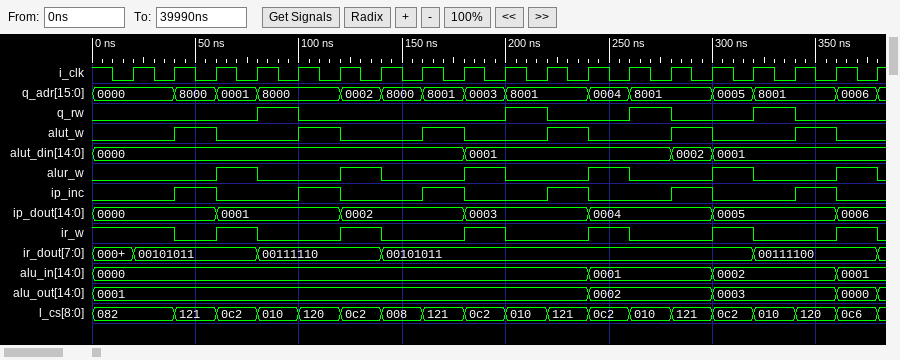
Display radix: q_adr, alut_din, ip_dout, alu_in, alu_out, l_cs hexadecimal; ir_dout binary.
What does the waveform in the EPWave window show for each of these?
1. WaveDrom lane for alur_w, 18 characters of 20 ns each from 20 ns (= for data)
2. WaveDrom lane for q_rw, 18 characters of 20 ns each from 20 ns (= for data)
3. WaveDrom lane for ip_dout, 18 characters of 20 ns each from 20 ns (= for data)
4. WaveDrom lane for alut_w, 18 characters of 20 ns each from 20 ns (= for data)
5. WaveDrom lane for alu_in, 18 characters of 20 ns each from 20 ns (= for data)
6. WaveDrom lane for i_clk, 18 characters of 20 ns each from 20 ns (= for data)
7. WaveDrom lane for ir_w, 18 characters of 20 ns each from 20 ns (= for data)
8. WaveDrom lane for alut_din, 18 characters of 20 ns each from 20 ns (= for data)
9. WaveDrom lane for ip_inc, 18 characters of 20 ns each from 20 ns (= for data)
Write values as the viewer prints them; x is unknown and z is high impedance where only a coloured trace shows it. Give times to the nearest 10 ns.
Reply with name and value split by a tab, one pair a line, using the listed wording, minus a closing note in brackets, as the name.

WaveDrom lane for alur_w, 18 characters of 20 ns each from 20 ns	{name: 'alur_w', wave: '0.10.10.10.10.10.1'}
WaveDrom lane for q_rw, 18 characters of 20 ns each from 20 ns	{name: 'q_rw', wave: '0..10....10.10.10.'}
WaveDrom lane for ip_dout, 18 characters of 20 ns each from 20 ns	{name: 'ip_dout', wave: '=.=..=..=..=..=..=', data: '0000 0001 0002 0003 0004 0005 0006'}
WaveDrom lane for alut_w, 18 characters of 20 ns each from 20 ns	{name: 'alut_w', wave: '010.10.10.10.10.10'}
WaveDrom lane for alu_in, 18 characters of 20 ns each from 20 ns	{name: 'alu_in', wave: '=..........=..=..=', data: '0000 0001 0002 0001'}
WaveDrom lane for i_clk, 18 characters of 20 ns each from 20 ns	{name: 'i_clk', wave: 'p.................'}
WaveDrom lane for ir_w, 18 characters of 20 ns each from 20 ns	{name: 'ir_w', wave: '1010.10.10.10.10.1'}
WaveDrom lane for alut_din, 18 characters of 20 ns each from 20 ns	{name: 'alut_din', wave: '=.......=....==...', data: '0000 0001 0002 0001'}
WaveDrom lane for ip_inc, 18 characters of 20 ns each from 20 ns	{name: 'ip_inc', wave: '010.10.10.10.10.10'}
